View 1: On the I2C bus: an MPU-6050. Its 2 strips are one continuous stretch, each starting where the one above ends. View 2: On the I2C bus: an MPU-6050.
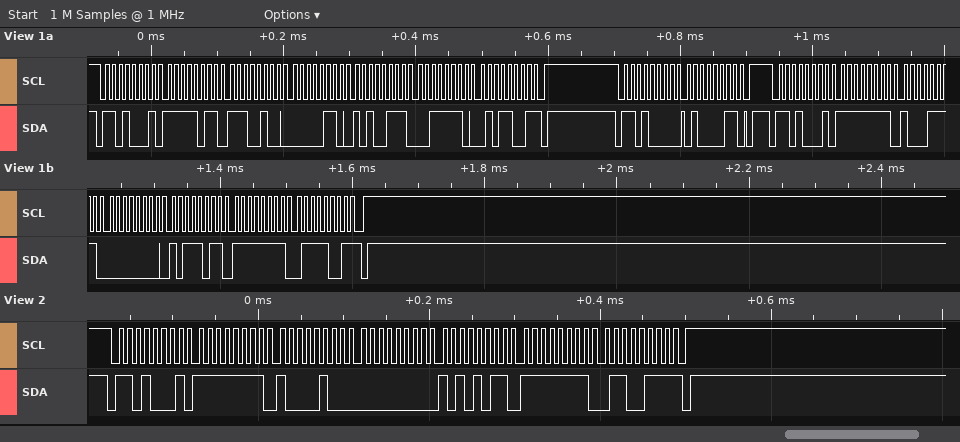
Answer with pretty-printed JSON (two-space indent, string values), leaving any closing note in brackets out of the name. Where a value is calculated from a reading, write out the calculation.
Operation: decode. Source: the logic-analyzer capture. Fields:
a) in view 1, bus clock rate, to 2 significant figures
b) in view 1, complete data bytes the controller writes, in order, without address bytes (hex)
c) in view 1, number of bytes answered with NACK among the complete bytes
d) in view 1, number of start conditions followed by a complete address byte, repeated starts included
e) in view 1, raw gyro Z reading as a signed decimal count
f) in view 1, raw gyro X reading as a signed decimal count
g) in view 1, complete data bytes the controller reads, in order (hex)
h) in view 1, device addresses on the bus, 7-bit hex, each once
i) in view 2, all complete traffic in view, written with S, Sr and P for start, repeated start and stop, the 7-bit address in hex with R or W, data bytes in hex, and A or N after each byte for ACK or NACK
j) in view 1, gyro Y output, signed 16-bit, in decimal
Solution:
{
  "in view 1, bus clock rate, to 2 significant figures": "100 kHz",
  "in view 1, complete data bytes the controller writes, in order, without address bytes": "43",
  "in view 1, number of bytes answered with NACK among the complete bytes": "2",
  "in view 1, number of start conditions followed by a complete address byte, repeated starts included": "3",
  "in view 1, raw gyro Z reading as a signed decimal count": "0xFF79 = -135",
  "in view 1, raw gyro X reading as a signed decimal count": "0xFF8F = -113",
  "in view 1, complete data bytes the controller reads, in order": "FB E4 06 A7 3E 59 FF 8F 00 BB FF 79",
  "in view 1, device addresses on the bus, 7-bit hex, each once": "0x68",
  "in view 2, all complete traffic in view, written with S, Sr and P for start, repeated start and stop, the 7-bit address in hex with R or W, data bytes in hex, and A or N after each byte for ACK or NACK": "S 68R A FF A 84 A 00 A AB A FF A 67 N P",
  "in view 1, gyro Y output, signed 16-bit, in decimal": "0x00BB = 187"
}
